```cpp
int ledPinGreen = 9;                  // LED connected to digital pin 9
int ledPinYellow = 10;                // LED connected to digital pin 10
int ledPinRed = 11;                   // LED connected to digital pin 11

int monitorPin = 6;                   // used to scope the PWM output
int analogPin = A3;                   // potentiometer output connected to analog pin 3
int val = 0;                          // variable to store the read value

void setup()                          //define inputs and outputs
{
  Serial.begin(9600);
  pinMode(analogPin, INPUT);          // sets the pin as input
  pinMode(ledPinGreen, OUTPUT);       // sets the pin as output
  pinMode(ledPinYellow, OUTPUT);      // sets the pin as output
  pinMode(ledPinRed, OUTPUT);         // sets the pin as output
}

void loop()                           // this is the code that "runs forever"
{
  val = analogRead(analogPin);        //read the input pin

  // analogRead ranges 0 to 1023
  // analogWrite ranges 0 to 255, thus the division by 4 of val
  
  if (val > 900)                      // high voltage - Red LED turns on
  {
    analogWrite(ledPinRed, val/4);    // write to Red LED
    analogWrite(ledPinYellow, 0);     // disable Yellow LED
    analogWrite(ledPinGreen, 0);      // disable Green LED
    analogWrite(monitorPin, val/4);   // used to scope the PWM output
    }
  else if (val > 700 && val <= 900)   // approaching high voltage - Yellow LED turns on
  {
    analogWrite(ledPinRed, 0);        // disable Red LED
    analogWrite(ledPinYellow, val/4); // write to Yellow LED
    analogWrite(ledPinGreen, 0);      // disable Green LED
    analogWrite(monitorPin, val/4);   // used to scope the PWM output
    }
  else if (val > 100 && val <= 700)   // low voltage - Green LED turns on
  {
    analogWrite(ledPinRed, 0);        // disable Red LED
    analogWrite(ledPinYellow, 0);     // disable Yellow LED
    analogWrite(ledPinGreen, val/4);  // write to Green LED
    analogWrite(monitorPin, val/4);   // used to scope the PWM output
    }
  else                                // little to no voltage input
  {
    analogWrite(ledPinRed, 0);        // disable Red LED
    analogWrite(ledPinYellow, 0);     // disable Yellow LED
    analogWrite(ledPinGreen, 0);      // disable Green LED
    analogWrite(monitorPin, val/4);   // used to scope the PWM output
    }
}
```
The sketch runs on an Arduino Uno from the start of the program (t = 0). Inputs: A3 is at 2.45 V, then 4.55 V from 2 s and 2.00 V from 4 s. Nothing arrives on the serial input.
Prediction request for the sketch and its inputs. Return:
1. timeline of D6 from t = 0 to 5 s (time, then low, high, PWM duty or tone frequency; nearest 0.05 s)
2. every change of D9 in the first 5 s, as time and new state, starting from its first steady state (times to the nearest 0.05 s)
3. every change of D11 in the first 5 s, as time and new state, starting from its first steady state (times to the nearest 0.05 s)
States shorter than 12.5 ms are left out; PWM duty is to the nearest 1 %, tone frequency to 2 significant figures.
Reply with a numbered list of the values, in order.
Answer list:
1. 0 s PWM 49 %; 2 s PWM 91 %; 4 s PWM 40 %
2. 0 s PWM 49 %; 2 s low; 4 s PWM 40 %
3. 0 s low; 2 s PWM 91 %; 4 s low
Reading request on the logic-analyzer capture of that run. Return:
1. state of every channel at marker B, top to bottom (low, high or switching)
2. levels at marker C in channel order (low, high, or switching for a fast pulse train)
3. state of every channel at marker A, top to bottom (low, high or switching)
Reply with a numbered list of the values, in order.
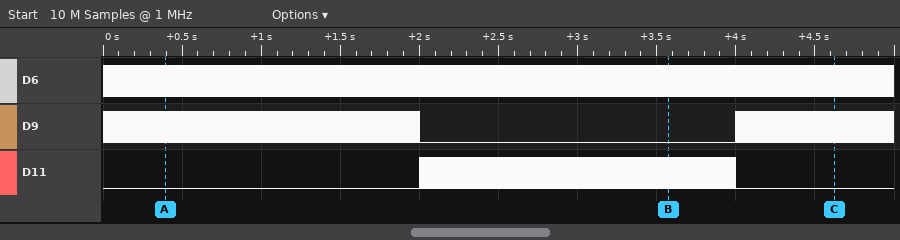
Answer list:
1. D6 switching, D9 low, D11 switching
2. D6 switching, D9 switching, D11 low
3. D6 switching, D9 switching, D11 low
